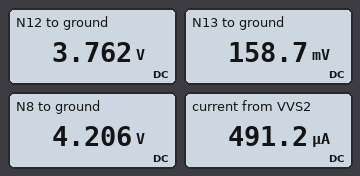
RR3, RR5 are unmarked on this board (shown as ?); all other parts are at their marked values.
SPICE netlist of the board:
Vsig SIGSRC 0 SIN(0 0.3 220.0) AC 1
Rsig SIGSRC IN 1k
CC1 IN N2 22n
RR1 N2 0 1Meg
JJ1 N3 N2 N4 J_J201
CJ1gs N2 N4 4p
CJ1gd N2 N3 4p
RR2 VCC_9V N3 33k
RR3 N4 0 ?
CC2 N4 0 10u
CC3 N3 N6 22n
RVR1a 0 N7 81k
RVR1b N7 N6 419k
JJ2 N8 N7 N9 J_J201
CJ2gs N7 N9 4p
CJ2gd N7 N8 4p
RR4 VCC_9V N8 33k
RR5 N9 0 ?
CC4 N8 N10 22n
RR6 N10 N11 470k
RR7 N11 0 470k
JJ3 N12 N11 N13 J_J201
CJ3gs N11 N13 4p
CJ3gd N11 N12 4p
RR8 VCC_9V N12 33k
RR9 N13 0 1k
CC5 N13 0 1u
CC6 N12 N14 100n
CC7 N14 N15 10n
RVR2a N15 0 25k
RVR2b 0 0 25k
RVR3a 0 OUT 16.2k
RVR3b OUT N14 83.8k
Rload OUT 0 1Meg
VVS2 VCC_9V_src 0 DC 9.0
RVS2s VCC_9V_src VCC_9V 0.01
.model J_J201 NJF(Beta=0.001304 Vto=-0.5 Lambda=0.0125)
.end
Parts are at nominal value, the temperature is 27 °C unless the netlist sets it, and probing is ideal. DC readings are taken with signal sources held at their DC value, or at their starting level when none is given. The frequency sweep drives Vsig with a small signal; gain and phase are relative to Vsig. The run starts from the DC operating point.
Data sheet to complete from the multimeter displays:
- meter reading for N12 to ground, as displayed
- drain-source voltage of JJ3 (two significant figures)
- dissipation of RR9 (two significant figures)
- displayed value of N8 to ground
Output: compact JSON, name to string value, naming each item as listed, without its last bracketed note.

{"meter reading for N12 to ground, as displayed": "3.762 V", "drain-source voltage of JJ3": "3.6 V", "dissipation of RR9": "25 µW", "displayed value of N8 to ground": "4.206 V"}
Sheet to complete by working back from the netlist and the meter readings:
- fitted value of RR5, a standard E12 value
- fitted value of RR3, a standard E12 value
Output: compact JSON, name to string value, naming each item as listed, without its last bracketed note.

{"fitted value of RR5, a standard E12 value": "1.2 kΩ", "fitted value of RR3, a standard E12 value": "680 Ω"}
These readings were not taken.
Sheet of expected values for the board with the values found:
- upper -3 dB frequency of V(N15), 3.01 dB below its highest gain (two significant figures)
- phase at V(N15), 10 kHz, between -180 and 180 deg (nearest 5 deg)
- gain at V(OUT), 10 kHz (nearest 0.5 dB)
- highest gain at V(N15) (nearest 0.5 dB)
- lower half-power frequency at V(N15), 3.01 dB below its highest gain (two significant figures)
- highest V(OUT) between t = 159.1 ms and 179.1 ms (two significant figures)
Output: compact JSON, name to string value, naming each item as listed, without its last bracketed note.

{"upper -3 dB frequency of V(N15), 3.01 dB below its highest gain": "12 kHz", "phase at V(N15), 10 kHz, between -180 and 180 deg": "130 deg", "gain at V(OUT), 10 kHz": "32.5 dB", "highest gain at V(N15)": "50.5 dB", "lower half-power frequency at V(N15), 3.01 dB below its highest gain": "430 Hz", "highest V(OUT) between t = 159.1 ms and 179.1 ms": "580 mV"}
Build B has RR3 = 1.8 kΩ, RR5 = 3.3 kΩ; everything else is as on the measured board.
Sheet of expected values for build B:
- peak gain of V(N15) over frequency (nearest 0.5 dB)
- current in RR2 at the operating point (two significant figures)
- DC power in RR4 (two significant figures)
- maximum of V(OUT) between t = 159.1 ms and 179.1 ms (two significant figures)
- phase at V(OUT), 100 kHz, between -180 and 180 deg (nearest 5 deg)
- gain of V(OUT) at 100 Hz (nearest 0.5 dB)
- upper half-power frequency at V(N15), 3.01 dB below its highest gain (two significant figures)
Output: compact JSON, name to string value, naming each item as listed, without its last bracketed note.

{"peak gain of V(N15) over frequency": "42.5 dB", "current in RR2 at the operating point": "120 µA", "DC power in RR4": "210 µW", "maximum of V(OUT) between t = 159.1 ms and 179.1 ms": "550 mV", "phase at V(OUT), 100 kHz, between -180 and 180 deg": "35 deg", "gain of V(OUT) at 100 Hz": "27.5 dB", "upper half-power frequency at V(N15), 3.01 dB below its highest gain": "13 kHz"}
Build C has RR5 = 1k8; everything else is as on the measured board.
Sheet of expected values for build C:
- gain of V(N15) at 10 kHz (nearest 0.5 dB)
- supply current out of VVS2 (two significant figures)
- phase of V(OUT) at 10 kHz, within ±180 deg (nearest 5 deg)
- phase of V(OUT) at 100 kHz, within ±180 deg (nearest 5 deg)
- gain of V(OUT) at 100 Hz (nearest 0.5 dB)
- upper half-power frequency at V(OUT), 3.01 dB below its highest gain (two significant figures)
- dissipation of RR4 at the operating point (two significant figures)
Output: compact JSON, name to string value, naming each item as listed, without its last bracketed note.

{"gain of V(N15) at 10 kHz": "46.0 dB", "supply current out of VVS2": "460 µA", "phase of V(OUT) at 10 kHz, within ±180 deg": "130 deg", "phase of V(OUT) at 100 kHz, within ±180 deg": "25 deg", "gain of V(OUT) at 100 Hz": "32.5 dB", "upper half-power frequency at V(OUT), 3.01 dB below its highest gain": "6.8 kHz", "dissipation of RR4 at the operating point": "450 µW"}
